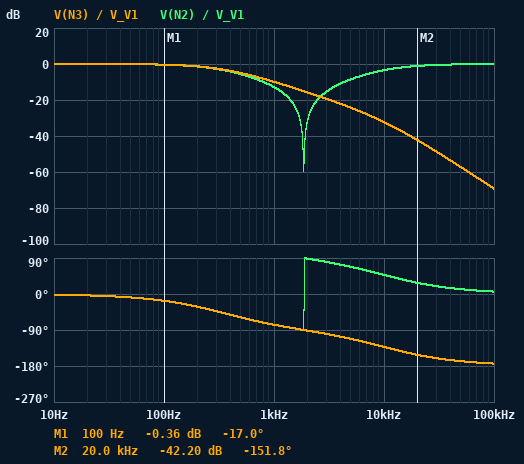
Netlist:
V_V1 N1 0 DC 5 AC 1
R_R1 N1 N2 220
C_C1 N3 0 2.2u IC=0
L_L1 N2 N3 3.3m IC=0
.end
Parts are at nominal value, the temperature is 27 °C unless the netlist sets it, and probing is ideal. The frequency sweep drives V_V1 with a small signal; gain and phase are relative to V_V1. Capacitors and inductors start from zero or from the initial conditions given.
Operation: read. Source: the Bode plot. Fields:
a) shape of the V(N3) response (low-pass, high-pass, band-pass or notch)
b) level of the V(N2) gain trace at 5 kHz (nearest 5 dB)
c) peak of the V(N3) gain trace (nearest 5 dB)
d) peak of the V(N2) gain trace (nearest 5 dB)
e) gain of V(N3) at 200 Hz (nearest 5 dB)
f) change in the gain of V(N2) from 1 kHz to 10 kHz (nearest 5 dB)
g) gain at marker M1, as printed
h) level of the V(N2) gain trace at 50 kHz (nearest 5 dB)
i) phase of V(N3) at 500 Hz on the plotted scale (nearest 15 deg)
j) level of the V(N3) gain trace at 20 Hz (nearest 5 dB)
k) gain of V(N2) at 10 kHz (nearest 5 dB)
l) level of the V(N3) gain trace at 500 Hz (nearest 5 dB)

low-pass
-10 dB
0 dB
0 dB
0 dB
10 dB
-0.36 dB
0 dB
-60 deg
0 dB
-5 dB
-5 dB
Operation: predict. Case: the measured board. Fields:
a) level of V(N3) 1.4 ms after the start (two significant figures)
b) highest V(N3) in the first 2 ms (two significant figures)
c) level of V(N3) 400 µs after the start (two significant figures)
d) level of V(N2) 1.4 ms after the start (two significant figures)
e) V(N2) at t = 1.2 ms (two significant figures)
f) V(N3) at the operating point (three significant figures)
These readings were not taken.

4.7 V
4.9 V
2.8 V
4.7 V
4.6 V
5.00 V
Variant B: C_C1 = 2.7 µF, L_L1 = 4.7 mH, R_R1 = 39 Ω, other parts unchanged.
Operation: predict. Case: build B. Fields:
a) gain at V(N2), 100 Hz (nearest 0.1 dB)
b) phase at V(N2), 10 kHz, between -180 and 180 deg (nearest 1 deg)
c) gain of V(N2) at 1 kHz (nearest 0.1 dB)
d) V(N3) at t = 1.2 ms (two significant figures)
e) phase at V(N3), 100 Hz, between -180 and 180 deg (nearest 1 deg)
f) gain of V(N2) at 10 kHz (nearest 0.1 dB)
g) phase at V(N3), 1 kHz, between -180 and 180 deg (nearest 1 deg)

0 dB
8 deg
-4.4 dB
5.0 V
-4 deg
-0.1 dB
-53 deg
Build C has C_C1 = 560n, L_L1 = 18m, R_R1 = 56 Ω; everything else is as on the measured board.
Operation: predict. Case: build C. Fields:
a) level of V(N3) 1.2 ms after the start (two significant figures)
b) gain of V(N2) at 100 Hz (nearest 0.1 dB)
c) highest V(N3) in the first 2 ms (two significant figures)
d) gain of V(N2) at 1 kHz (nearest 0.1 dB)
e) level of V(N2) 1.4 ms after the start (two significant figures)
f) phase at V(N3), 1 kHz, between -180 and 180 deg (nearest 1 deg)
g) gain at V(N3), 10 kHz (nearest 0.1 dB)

4.5 V
0 dB
8.0 V
-0.4 dB
4.8 V
-18 deg
-31.8 dB
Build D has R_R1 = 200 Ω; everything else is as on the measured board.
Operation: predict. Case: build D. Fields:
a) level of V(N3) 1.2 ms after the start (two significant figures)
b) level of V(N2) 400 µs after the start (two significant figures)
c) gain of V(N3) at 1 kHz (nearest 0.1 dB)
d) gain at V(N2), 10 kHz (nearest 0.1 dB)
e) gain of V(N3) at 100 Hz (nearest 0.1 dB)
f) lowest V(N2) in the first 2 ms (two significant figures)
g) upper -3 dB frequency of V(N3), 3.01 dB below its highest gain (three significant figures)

4.7 V
2.9 V
-9.1 dB
-3.0 dB
-0.3 dB
460 mV
376 Hz
